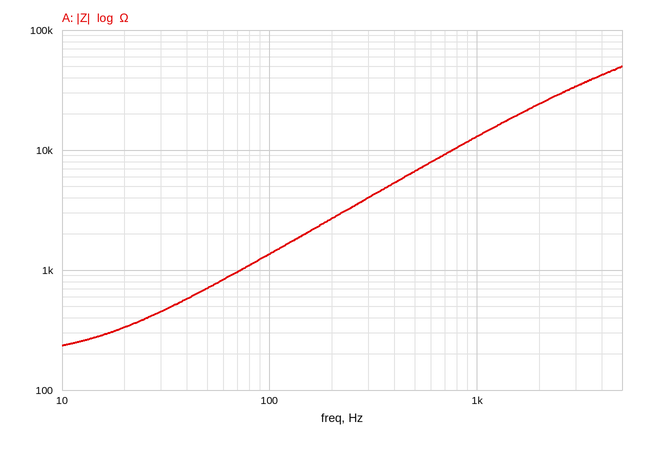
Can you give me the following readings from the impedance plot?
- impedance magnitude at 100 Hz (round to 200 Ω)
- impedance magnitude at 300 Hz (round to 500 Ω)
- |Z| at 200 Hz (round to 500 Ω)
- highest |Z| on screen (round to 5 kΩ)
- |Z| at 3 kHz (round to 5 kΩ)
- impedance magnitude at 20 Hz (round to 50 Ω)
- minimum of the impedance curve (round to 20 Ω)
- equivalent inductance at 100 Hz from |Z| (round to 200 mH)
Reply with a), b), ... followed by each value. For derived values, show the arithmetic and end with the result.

a) 1.4 kΩ
b) 4.0 kΩ
c) 2.5 kΩ
d) 50 kΩ
e) 35 kΩ
f) 350 Ω
g) 240 Ω
h) L = 1.4 kΩ/(2π × 100 Hz) ≈ 2.2 H
